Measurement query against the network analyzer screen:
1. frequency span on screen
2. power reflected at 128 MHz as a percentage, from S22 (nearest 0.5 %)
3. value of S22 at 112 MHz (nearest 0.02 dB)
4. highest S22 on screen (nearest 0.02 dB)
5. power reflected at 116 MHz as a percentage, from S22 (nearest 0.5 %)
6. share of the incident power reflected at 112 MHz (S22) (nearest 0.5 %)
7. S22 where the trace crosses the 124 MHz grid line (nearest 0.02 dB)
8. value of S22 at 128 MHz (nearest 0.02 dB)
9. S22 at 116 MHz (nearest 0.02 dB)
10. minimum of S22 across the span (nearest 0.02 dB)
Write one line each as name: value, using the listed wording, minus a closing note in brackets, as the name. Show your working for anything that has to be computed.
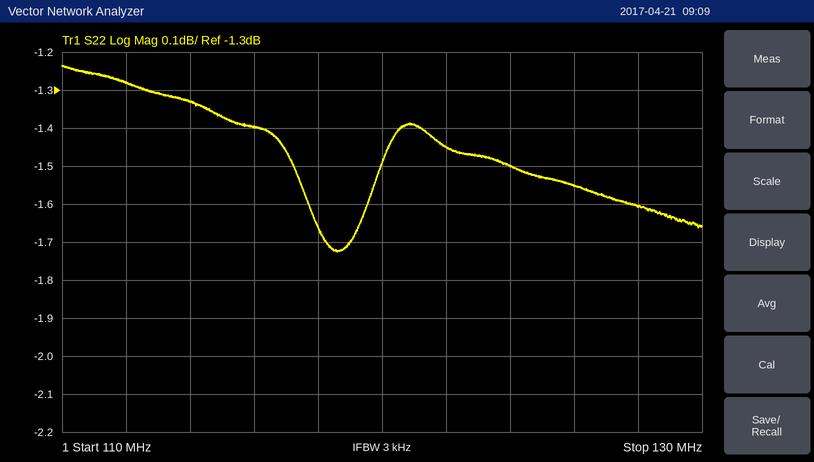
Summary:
frequency span on screen: 20 MHz
power reflected at 128 MHz as a percentage, from S22: 10^(-1.6/10) ≈ 69.2 %, so 69.0 % to the nearest 0.5 %
value of S22 at 112 MHz: -1.28 dB
highest S22 on screen: -1.24 dB
power reflected at 116 MHz as a percentage, from S22: 10^(-1.4/10) ≈ 72.4 %, so 72.5 % to the nearest 0.5 %
share of the incident power reflected at 112 MHz (S22): 10^(-1.28/10) ≈ 74.5 %
S22 where the trace crosses the 124 MHz grid line: -1.50 dB
value of S22 at 128 MHz: -1.60 dB
S22 at 116 MHz: -1.40 dB
minimum of S22 across the span: -1.72 dB
